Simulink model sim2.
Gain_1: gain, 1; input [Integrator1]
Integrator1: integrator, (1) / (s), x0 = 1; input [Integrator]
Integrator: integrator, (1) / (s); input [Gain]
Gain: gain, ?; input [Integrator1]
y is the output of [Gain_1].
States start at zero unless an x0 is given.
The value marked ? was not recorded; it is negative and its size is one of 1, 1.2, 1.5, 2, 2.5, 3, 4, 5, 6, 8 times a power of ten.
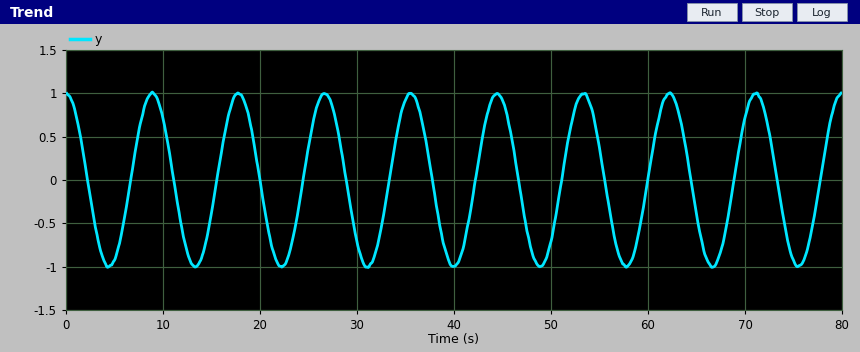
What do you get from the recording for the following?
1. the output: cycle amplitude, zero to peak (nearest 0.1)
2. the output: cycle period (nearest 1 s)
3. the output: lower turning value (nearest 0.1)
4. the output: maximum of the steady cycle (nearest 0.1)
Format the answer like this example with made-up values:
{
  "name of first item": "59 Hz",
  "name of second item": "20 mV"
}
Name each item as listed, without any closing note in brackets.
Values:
{
  "the output: cycle amplitude, zero to peak": "1.0",
  "the output: cycle period": "9 s",
  "the output: lower turning value": "-1.0",
  "the output: maximum of the steady cycle": "1.0"
}
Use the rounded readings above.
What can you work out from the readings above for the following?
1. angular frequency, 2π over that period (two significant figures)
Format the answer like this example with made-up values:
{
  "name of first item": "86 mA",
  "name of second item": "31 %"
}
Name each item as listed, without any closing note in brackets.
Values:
{
  "angular frequency, 2π over that period": "0.70 rad/s"
}
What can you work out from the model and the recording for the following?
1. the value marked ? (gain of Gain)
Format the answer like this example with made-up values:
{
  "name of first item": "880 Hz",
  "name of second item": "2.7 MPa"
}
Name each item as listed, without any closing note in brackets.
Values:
{
  "the value marked ?": "-0.5"
}
